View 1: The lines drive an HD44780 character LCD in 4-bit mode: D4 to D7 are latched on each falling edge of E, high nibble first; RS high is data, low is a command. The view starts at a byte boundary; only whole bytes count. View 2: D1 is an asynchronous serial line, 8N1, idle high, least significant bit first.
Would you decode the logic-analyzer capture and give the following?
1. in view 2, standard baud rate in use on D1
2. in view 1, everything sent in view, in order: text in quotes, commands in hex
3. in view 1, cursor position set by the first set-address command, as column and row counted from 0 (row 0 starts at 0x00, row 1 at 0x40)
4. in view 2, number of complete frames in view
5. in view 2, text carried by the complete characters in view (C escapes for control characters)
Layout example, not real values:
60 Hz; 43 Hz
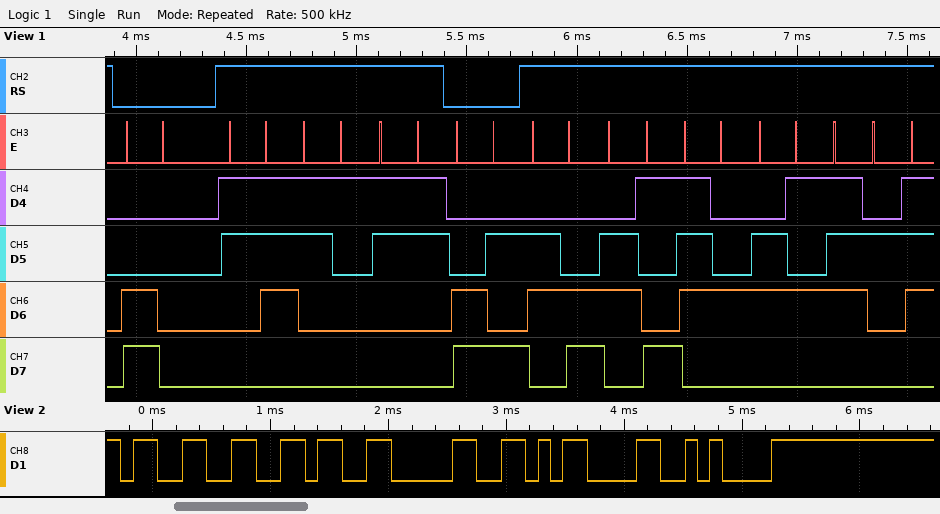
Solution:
9600 baud; 0xC0 "713" 0xCA "liter"; column 0, row 1; 5; "360\r\n"
